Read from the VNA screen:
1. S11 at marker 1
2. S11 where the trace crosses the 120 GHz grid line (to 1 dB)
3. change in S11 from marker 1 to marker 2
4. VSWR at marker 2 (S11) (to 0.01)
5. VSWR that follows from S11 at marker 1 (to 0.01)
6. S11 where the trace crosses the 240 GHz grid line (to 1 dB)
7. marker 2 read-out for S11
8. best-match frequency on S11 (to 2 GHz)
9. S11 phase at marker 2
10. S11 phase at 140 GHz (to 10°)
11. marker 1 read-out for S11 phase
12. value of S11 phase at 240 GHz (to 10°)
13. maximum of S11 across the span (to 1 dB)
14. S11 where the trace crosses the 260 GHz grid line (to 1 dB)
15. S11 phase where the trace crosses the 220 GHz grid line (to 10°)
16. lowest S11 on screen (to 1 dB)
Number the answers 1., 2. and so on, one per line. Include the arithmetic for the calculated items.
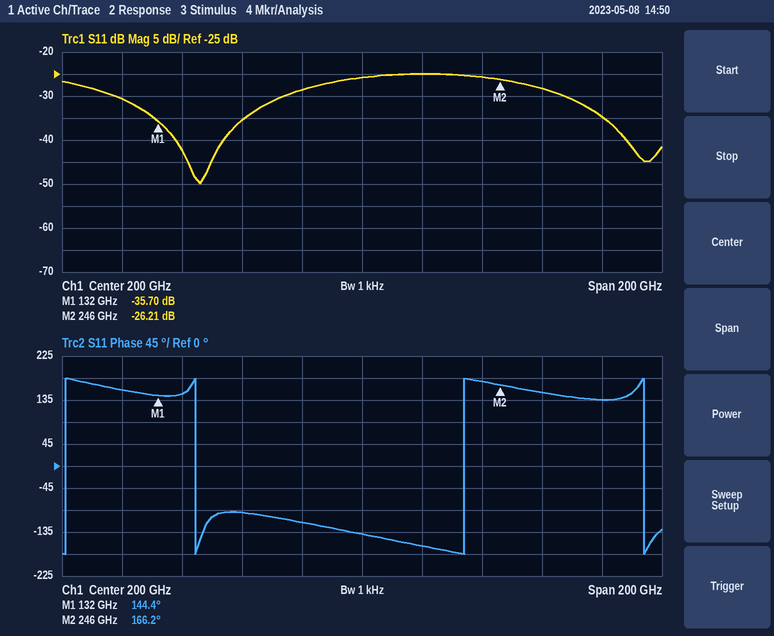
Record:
1. -35.70 dB
2. -31 dB
3. -26.21 − (-35.7) = 9.49 dB
4. (1 + 0.0489)/(1 − 0.0489) ≈ 1.10
5. (1 + 0.0164)/(1 − 0.0164) ≈ 1.03
6. -26 dB
7. -26.21 dB
8. 146 GHz
9. 166.2°
10. 150°
11. 144.4°
12. 170°
13. -25 dB
14. -28 dB
15. -160°
16. -50 dB
